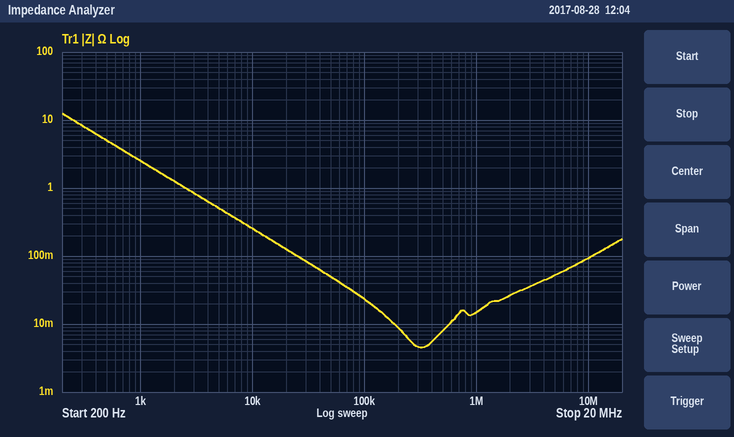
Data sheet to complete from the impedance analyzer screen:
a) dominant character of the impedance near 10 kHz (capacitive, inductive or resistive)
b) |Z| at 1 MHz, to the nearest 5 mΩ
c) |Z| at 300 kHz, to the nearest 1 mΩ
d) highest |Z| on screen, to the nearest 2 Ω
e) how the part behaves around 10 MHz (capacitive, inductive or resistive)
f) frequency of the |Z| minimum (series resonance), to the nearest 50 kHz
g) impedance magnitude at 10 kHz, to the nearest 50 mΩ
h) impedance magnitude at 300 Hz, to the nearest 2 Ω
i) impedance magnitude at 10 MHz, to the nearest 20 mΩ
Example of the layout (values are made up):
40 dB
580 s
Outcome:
capacitive
15 mΩ
5 mΩ
12 Ω
inductive
300 kHz
250 mΩ
8 Ω
100 mΩ
